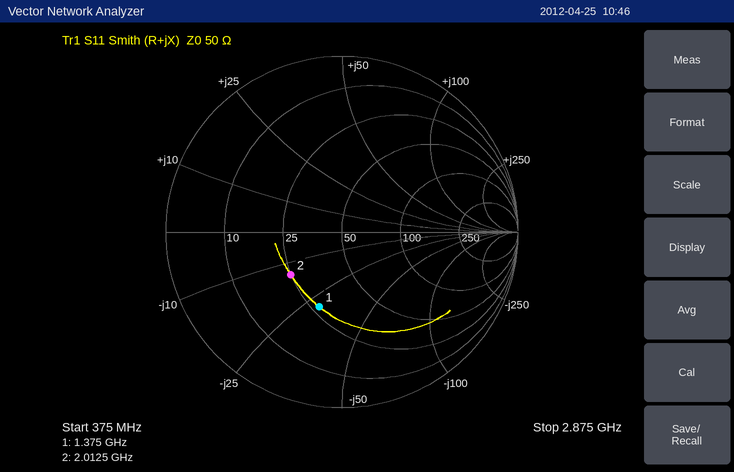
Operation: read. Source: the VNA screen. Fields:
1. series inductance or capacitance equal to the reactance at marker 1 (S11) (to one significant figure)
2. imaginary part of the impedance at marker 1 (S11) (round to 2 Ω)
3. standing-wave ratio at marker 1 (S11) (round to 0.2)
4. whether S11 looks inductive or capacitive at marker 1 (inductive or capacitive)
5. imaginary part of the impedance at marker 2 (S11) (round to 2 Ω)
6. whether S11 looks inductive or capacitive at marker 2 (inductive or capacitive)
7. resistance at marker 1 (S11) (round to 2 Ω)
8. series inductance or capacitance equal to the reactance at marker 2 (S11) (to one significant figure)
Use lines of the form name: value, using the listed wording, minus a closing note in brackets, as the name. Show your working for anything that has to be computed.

series inductance or capacitance equal to the reactance at marker 1 (S11): C = 1/(2π × 1.375 GHz × 30 Ω) ≈ 4 pF
imaginary part of the impedance at marker 1 (S11): -30 Ω
standing-wave ratio at marker 1 (S11): 2.6
whether S11 looks inductive or capacitive at marker 1: capacitive
imaginary part of the impedance at marker 2 (S11): -14 Ω
whether S11 looks inductive or capacitive at marker 2: capacitive
resistance at marker 1 (S11): 28 Ω
series inductance or capacitance equal to the reactance at marker 2 (S11): C = 1/(2π × 2.0125 GHz × 14 Ω) ≈ 6 pF
